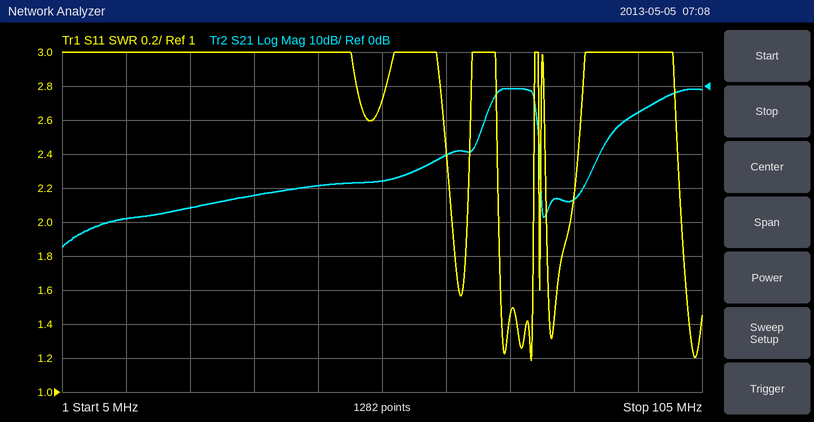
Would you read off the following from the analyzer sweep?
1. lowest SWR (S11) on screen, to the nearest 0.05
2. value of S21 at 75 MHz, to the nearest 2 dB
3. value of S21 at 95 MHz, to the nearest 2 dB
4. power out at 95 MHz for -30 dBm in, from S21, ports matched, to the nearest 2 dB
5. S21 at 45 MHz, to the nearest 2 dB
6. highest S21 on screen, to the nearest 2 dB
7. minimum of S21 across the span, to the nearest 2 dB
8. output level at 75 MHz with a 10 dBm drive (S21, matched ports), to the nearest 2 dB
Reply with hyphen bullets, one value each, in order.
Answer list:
- 1.20
- 0 dB
- -8 dB
- -38 dBm
- -30 dB
- 0 dB
- -48 dB
- 10 dBm
